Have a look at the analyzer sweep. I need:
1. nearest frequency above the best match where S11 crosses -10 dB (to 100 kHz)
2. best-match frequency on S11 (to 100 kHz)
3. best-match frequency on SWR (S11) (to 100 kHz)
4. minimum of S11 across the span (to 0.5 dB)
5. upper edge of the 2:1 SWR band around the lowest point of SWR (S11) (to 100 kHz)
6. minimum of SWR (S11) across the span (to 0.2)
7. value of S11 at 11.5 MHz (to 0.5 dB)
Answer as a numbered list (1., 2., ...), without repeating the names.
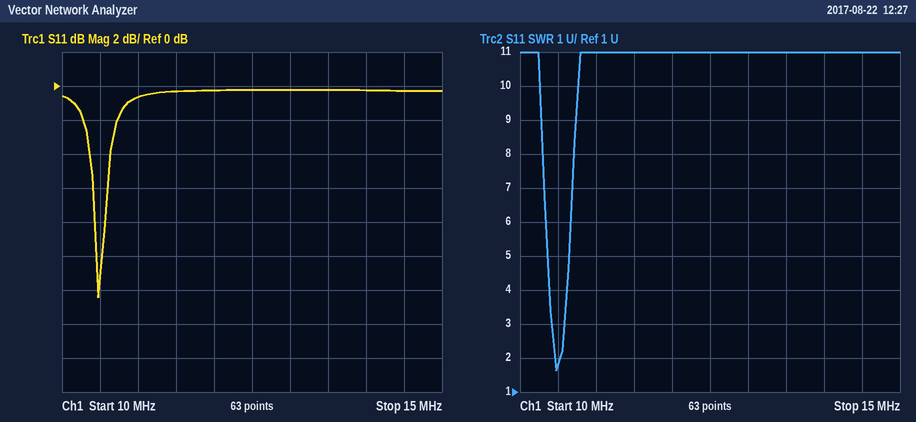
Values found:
1. 10.5 MHz
2. 10.5 MHz
3. 10.5 MHz
4. -12.5 dB
5. 10.5 MHz
6. 1.6
7. -0.5 dB
